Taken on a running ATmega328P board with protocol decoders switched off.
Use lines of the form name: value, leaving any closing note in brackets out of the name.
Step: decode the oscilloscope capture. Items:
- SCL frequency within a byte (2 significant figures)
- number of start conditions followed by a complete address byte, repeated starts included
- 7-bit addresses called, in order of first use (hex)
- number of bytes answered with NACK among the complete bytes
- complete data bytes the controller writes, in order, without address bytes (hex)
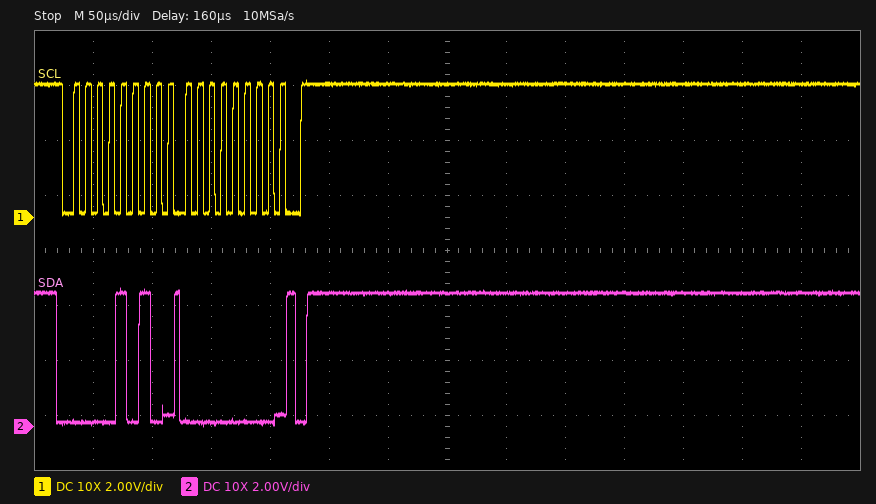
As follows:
SCL frequency within a byte: 100 kHz
number of start conditions followed by a complete address byte, repeated starts included: 1
7-bit addresses called, in order of first use: 0x05
number of bytes answered with NACK among the complete bytes: 0
complete data bytes the controller writes, in order, without address bytes: 00
